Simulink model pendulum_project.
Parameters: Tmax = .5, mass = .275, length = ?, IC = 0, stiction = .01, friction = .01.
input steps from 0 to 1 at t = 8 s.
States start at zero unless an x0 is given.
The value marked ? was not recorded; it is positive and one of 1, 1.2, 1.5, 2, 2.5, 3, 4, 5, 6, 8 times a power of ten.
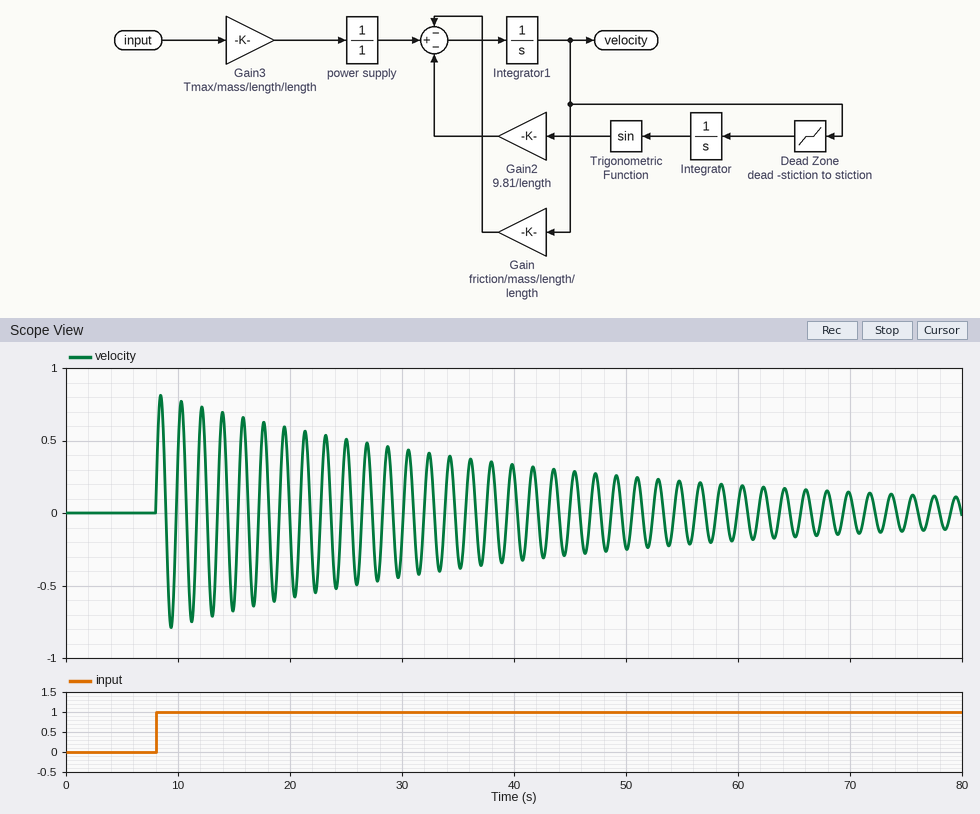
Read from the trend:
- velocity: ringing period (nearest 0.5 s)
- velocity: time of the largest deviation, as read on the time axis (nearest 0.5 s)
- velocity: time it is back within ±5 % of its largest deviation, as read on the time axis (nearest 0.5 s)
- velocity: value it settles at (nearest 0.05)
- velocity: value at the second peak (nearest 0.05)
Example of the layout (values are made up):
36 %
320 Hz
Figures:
2.0 s
8.5 s
80.0 s
0.00
0.75
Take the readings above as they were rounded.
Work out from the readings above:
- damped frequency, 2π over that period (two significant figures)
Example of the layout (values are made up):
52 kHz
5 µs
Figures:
3.1 rad/s
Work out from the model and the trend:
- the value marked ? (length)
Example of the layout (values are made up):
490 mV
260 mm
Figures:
0.8
